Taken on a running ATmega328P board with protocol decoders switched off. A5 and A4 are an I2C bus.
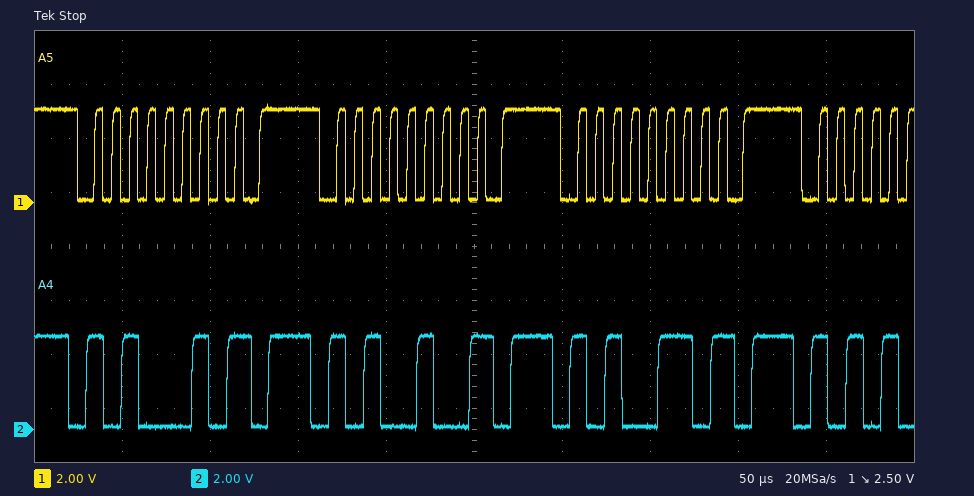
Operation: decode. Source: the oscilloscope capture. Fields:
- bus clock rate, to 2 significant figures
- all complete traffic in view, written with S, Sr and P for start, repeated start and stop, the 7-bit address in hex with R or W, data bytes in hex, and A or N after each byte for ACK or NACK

100 kHz
S 51W N P S 52W N P S 53W N P
